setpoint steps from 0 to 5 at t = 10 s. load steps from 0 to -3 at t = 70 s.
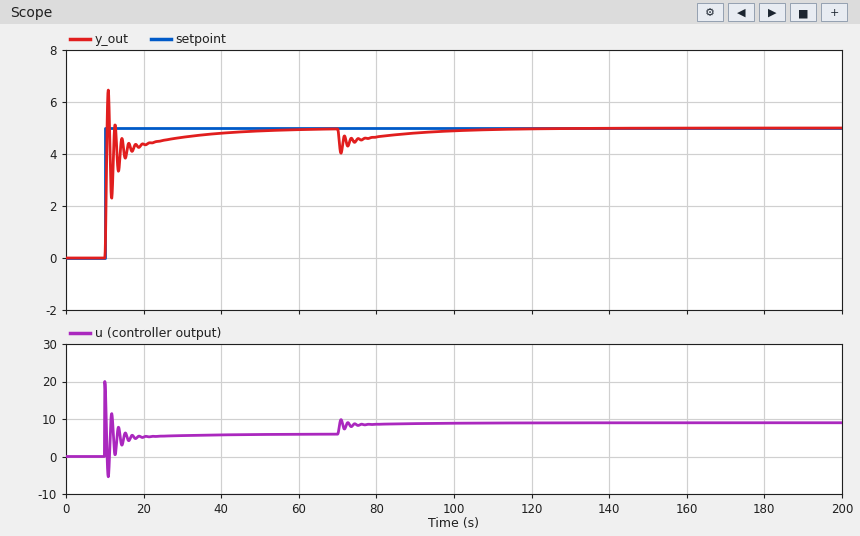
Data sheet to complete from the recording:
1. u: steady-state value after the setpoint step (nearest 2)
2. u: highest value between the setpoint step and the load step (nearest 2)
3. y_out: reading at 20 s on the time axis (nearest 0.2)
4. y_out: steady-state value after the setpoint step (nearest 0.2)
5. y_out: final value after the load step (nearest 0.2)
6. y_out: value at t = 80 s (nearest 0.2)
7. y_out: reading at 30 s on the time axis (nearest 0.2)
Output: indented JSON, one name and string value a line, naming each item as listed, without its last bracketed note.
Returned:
{
  "u: steady-state value after the setpoint step": "6",
  "u: highest value between the setpoint step and the load step": "20",
  "y_out: reading at 20 s on the time axis": "4.4",
  "y_out: steady-state value after the setpoint step": "5.0",
  "y_out: final value after the load step": "5.0",
  "y_out: value at t = 80 s": "4.6",
  "y_out: reading at 30 s on the time axis": "4.6"
}
